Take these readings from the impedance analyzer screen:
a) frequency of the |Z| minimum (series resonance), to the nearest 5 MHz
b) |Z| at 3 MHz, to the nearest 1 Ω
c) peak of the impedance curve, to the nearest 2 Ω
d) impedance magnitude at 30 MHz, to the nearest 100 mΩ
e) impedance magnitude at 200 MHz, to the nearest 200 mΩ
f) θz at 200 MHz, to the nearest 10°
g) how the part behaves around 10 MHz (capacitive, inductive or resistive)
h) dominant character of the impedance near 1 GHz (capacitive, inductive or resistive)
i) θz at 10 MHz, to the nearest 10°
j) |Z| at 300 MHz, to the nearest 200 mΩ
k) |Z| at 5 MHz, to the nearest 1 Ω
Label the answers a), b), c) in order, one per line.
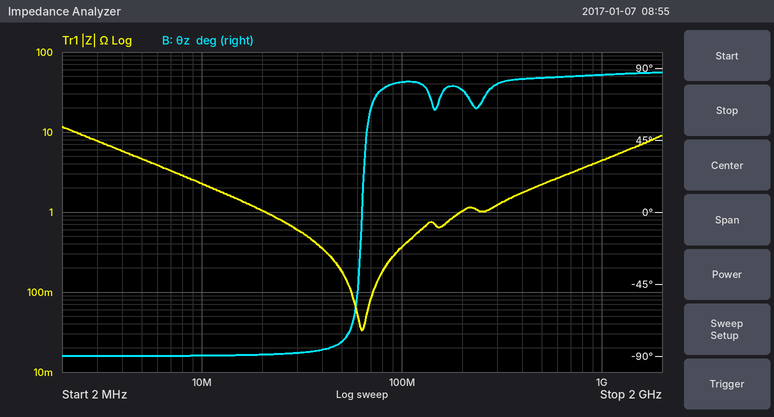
a) 65 MHz
b) 8 Ω
c) 12 Ω
d) 600 mΩ
e) 1.0 Ω
f) 80°
g) capacitive
h) inductive
i) -90°
j) 1.2 Ω
k) 5 Ω
